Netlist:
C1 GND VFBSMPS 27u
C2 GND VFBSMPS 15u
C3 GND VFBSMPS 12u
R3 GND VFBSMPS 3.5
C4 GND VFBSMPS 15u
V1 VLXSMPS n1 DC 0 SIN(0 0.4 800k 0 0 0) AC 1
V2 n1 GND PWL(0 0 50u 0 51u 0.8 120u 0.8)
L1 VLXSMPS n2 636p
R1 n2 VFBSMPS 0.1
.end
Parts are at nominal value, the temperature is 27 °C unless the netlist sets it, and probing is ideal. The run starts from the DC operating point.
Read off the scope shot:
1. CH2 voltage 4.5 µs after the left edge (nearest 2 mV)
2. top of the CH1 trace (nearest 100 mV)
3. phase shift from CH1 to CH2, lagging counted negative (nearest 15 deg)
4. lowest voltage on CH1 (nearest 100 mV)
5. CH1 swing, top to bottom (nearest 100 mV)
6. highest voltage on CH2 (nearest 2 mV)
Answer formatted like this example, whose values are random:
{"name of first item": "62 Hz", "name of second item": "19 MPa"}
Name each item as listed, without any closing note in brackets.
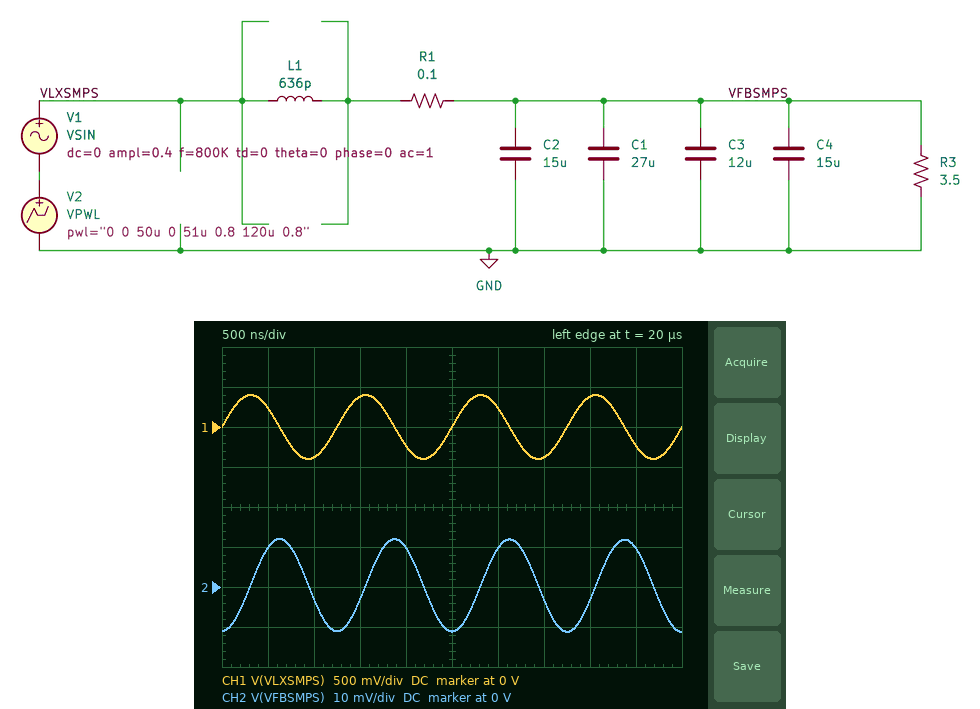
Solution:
{"CH2 voltage 4.5 µs after the left edge": "10 mV", "top of the CH1 trace": "400 mV", "phase shift from CH1 to CH2, lagging counted negative": "-90 deg", "lowest voltage on CH1": "-400 mV", "CH1 swing, top to bottom": "800 mV", "highest voltage on CH2": "12 mV"}
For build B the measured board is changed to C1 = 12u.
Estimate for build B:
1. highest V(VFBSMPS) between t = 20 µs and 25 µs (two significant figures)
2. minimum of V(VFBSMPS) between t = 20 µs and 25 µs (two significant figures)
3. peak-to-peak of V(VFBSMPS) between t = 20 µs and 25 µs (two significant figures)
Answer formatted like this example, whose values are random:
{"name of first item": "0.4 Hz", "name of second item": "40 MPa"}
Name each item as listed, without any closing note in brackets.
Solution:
{"highest V(VFBSMPS) between t = 20 µs and 25 µs": "15 mV", "minimum of V(VFBSMPS) between t = 20 µs and 25 µs": "-15 mV", "peak-to-peak of V(VFBSMPS) between t = 20 µs and 25 µs": "30 mV"}
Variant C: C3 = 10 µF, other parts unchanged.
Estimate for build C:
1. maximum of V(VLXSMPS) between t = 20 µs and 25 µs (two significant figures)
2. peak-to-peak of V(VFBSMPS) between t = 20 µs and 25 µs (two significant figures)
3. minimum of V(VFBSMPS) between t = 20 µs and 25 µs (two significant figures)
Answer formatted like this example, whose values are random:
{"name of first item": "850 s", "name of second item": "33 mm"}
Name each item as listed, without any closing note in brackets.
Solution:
{"maximum of V(VLXSMPS) between t = 20 µs and 25 µs": "400 mV", "peak-to-peak of V(VFBSMPS) between t = 20 µs and 25 µs": "24 mV", "minimum of V(VFBSMPS) between t = 20 µs and 25 µs": "-12 mV"}
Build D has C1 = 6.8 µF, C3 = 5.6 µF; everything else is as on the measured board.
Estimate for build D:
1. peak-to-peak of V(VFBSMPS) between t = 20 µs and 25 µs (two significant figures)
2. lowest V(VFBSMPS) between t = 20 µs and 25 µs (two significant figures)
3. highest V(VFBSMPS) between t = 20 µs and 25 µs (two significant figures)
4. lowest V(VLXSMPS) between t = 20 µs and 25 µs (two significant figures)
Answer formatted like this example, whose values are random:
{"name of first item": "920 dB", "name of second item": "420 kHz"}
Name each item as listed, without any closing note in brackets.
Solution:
{"peak-to-peak of V(VFBSMPS) between t = 20 µs and 25 µs": "38 mV", "lowest V(VFBSMPS) between t = 20 µs and 25 µs": "-19 mV", "highest V(VFBSMPS) between t = 20 µs and 25 µs": "19 mV", "lowest V(VLXSMPS) between t = 20 µs and 25 µs": "-400 mV"}
